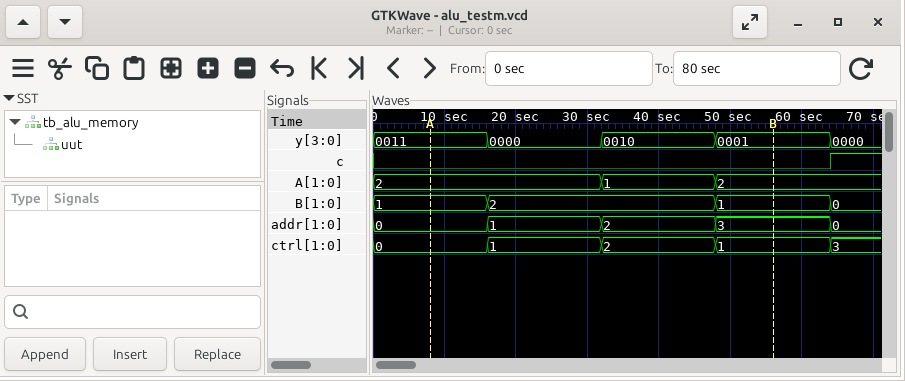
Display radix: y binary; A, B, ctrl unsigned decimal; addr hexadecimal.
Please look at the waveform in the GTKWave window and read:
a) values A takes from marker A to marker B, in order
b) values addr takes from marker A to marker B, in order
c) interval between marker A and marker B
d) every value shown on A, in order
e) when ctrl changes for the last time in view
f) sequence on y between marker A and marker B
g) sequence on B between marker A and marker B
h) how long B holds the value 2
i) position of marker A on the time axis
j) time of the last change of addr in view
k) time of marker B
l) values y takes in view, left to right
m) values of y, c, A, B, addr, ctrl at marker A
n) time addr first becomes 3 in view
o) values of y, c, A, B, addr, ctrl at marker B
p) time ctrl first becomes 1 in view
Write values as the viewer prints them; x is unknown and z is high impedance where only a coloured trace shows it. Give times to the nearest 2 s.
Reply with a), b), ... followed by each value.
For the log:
a) 2, 1, 2
b) 0, 1, 2, 3
c) 48 s
d) 2, 1, 2
e) 64 s
f) 0011, 0000, 0010, 0001
g) 1, 2, 1
h) 32 s
i) 8 s
j) 64 s
k) 56 s
l) 0011, 0000, 0010, 0001, 0000
m) y=0011, c=0, A=2, B=1, addr=0, ctrl=0
n) 48 s
o) y=0001, c=0, A=2, B=1, addr=3, ctrl=1
p) 16 s
